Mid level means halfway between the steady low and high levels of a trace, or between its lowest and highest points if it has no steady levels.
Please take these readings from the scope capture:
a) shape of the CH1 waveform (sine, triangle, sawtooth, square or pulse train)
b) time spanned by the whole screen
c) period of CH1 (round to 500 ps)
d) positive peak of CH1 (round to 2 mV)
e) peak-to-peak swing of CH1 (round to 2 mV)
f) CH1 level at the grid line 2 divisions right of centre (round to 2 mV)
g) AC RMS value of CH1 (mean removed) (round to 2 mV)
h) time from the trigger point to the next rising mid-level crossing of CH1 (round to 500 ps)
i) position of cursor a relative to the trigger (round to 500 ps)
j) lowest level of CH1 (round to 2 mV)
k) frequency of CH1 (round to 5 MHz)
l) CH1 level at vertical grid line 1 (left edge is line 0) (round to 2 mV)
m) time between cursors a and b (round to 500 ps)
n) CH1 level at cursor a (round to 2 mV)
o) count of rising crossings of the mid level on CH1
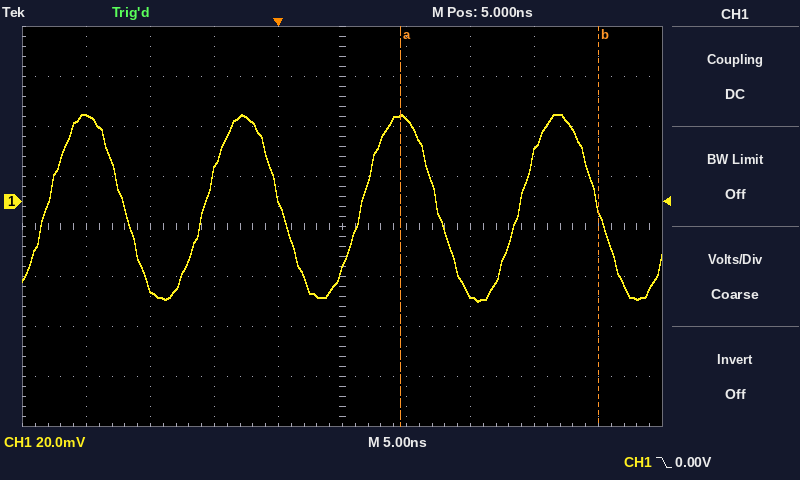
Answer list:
sine
50 ns
12.5 ns
34 mV
74 mV
-38 mV
26 mV
6.5 ns
+9.5 ns
-40 mV
80 MHz
34 mV
15.5 ns
34 mV
4
